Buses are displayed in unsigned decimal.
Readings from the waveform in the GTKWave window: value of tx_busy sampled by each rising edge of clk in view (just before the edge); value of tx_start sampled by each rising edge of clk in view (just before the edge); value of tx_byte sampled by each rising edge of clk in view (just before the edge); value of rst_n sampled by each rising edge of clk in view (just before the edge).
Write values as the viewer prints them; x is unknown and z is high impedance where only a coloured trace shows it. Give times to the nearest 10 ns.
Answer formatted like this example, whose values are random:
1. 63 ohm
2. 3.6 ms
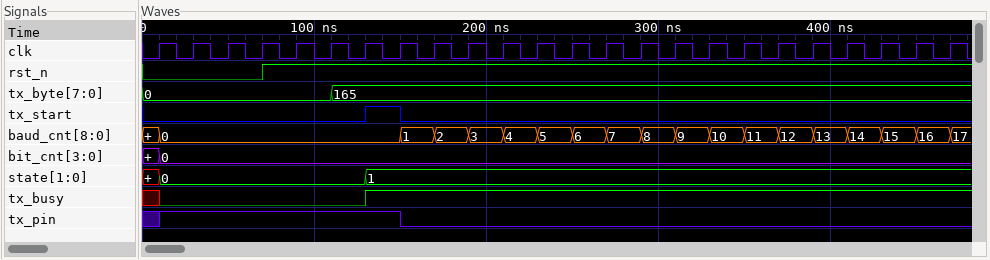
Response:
1. x 0 0 0 0 0 0 1 1 1 1 1 1 1 1 1 1 1 1 1 1 1 1 1
2. 0 0 0 0 0 0 0 1 0 0 0 0 0 0 0 0 0 0 0 0 0 0 0 0
3. 0, 0, 0, 0, 0, 0, 165, 165, 165, 165, 165, 165, 165, 165, 165, 165, 165, 165, 165, 165, 165, 165, 165, 165
4. 0 0 0 0 1 1 1 1 1 1 1 1 1 1 1 1 1 1 1 1 1 1 1 1
